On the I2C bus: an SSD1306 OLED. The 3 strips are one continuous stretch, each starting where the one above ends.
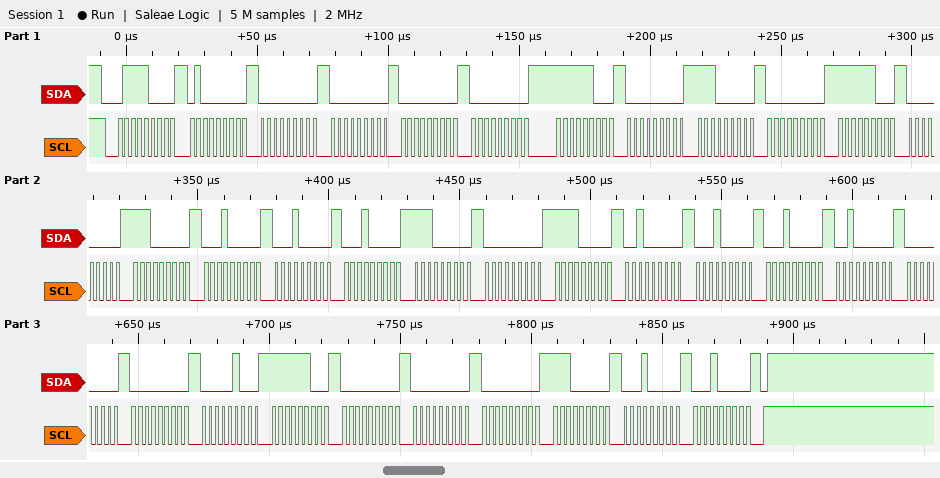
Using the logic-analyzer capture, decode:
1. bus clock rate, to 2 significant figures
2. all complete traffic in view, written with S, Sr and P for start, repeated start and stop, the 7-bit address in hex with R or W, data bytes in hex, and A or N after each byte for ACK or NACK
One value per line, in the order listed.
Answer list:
400 kHz
S 3CW A 40 A 00 A 00 A 00 A 00 A FC A 00 A E0 A 00 A FC A 00 A E0 A 10 A 10 A 10 A E0 A 00 A F0 A 20 A 10 A 10 A 20 A 00 A 00 A 04 A FC A 00 A 00 A 00 A E0 A 10 A 10 A P
